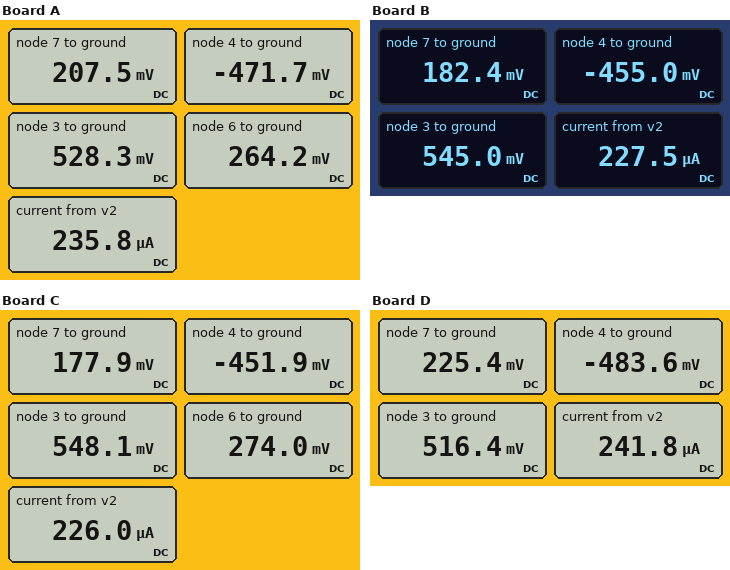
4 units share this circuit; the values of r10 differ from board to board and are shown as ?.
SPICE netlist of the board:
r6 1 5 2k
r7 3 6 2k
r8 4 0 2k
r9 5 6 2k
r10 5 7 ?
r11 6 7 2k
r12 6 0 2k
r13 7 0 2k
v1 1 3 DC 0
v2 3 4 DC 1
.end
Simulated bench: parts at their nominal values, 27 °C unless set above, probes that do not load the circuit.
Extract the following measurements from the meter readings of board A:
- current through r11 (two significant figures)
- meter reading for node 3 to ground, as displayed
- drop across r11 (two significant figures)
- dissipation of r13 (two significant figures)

28 µA
528.3 mV
57 mV
22 µW
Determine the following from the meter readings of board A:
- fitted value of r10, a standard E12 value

1.5 kΩ
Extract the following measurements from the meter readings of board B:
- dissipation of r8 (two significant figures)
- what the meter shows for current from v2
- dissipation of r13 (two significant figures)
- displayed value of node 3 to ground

100 µW
227.5 µA
17 µW
545.0 mV
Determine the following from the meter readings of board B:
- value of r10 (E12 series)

3.9 kΩ
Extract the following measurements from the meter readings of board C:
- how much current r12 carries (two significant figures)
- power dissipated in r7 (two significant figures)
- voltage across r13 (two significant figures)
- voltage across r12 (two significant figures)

140 µA
38 µW
180 mV
270 mV
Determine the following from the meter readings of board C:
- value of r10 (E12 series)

4.7 kΩ
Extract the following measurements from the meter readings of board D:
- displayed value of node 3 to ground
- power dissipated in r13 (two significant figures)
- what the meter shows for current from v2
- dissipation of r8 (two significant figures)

516.4 mV
25 µW
241.8 µA
120 µW
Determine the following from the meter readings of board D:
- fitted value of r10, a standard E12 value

680 Ω
